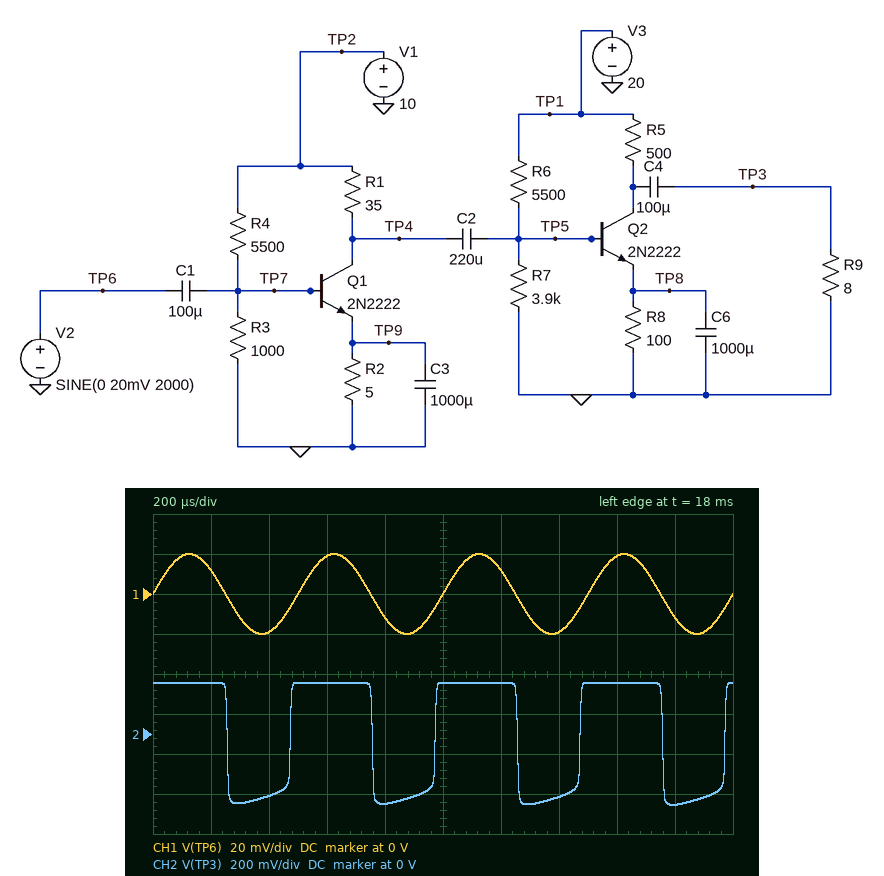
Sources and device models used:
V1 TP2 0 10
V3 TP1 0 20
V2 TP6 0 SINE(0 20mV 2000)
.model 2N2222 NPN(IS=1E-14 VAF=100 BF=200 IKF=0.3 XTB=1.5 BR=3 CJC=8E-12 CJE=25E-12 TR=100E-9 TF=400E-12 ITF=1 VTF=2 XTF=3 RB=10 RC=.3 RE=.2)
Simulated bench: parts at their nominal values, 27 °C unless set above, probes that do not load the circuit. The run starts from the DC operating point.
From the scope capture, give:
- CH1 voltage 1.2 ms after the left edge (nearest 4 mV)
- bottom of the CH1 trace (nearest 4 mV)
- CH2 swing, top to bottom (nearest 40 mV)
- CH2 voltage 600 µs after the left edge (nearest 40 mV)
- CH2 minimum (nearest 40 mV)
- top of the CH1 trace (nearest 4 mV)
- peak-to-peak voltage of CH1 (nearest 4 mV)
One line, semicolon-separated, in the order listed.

12 mV; -20 mV; 600 mV; 240 mV; -360 mV; 20 mV; 40 mV
